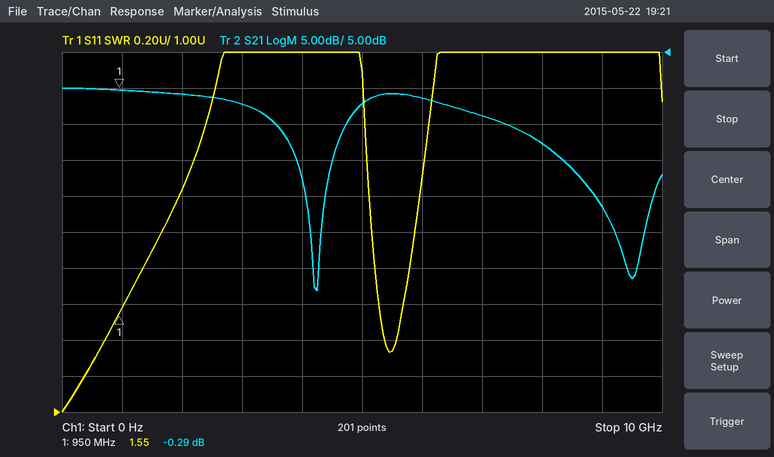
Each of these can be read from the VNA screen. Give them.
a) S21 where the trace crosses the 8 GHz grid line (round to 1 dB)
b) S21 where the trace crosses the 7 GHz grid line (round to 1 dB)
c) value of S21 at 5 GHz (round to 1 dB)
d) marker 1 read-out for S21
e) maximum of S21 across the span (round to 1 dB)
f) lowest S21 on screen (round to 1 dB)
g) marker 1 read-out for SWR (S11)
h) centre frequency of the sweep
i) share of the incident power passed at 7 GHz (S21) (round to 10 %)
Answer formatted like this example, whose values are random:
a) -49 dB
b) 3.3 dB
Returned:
a) -8 dB
b) -4 dB
c) -2 dB
d) -0.29 dB
e) 0 dB
f) -28 dB
g) 1.55
h) 5 GHz
i) 40 %
